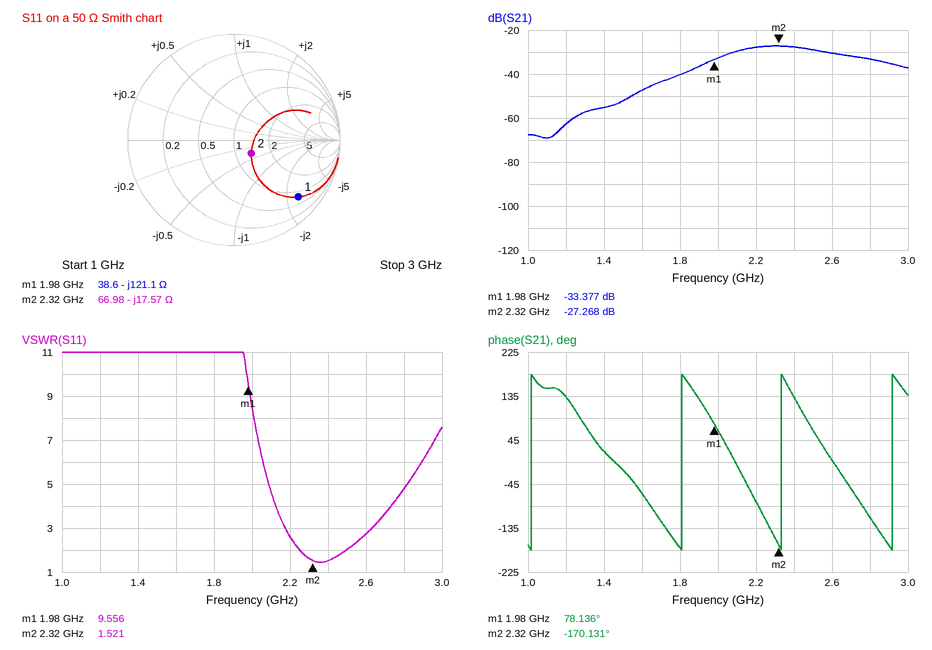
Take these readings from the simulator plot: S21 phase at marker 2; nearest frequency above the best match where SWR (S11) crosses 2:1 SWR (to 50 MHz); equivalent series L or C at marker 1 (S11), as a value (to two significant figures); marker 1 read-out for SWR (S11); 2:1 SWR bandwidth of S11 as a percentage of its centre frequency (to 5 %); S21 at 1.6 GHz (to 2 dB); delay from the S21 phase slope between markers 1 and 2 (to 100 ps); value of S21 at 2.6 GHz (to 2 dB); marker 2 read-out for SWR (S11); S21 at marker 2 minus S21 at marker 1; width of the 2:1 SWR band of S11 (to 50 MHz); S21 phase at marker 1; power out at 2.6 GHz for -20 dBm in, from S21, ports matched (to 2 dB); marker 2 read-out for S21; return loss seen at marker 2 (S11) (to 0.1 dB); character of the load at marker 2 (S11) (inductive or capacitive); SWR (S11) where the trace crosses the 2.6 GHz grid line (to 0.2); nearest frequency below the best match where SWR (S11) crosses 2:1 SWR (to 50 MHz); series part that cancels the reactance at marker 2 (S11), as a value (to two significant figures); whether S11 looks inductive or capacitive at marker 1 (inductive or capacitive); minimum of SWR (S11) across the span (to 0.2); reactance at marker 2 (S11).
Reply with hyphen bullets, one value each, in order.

- -170.131°
- 2.50 GHz
- 660 fF
- 9.556
- 10 %
- -48 dB
- 2.0 ns
- -30 dB
- 1.521
- 6.109 dB
- 250 MHz
- 78.136°
- -50 dBm
- -27.268 dB
- 13.7 dB
- capacitive
- 2.8
- 2.25 GHz
- 1.2 nH
- capacitive
- 1.4
- -17.57 Ω
